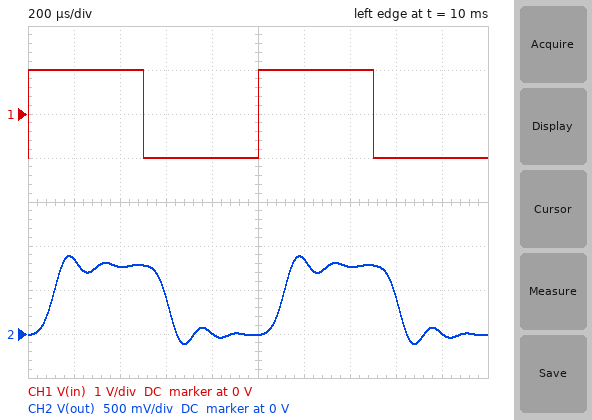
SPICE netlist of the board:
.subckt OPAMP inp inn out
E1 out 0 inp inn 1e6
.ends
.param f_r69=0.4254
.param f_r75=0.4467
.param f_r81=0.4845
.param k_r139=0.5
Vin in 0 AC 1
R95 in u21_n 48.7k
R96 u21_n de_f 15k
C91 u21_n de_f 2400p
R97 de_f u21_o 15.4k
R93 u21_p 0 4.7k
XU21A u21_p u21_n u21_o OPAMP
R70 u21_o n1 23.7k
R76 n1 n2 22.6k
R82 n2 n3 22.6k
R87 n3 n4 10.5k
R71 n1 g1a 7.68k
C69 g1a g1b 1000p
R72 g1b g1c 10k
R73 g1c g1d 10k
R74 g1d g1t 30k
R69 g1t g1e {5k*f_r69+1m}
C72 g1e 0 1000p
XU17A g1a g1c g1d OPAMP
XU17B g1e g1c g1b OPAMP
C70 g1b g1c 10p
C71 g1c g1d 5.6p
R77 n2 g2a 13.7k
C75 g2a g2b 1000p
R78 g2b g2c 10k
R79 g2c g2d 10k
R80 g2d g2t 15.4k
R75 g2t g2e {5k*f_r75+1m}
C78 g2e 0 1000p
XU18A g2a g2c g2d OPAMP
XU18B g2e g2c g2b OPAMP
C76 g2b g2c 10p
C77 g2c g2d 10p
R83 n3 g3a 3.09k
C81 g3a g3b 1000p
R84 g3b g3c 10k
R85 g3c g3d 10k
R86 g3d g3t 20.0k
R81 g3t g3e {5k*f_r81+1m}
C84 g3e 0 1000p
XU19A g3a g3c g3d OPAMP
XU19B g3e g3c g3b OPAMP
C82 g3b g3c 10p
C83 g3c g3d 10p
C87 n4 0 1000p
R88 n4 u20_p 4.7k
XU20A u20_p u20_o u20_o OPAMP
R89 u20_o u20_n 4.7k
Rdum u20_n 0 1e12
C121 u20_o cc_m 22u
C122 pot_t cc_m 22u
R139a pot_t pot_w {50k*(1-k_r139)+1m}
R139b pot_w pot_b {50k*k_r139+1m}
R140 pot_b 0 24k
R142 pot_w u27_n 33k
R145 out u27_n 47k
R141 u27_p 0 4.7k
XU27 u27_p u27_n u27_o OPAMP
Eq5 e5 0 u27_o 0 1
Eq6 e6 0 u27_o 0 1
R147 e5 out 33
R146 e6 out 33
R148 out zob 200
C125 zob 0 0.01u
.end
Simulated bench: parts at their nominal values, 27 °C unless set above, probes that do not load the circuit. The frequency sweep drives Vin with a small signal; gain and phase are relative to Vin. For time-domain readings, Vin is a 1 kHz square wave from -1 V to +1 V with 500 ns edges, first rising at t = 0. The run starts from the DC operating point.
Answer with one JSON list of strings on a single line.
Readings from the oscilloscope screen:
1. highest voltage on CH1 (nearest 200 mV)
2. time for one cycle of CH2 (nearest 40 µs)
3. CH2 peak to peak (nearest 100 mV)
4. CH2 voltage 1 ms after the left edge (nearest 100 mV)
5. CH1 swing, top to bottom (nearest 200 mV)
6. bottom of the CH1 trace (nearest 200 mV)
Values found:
["1.0 V", "1.00 ms", "1.0 V", "0 V", "2.0 V", "-1.0 V"]
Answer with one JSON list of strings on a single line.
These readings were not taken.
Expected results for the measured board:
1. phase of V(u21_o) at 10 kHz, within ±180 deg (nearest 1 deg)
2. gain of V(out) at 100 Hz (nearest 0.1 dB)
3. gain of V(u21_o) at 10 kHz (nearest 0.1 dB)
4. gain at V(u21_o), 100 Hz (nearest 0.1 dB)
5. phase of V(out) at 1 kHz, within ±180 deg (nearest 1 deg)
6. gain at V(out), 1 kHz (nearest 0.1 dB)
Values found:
["163 deg", "-8.1 dB", "-8.3 dB", "-4.1 dB", "-35 deg", "-8.3 dB"]
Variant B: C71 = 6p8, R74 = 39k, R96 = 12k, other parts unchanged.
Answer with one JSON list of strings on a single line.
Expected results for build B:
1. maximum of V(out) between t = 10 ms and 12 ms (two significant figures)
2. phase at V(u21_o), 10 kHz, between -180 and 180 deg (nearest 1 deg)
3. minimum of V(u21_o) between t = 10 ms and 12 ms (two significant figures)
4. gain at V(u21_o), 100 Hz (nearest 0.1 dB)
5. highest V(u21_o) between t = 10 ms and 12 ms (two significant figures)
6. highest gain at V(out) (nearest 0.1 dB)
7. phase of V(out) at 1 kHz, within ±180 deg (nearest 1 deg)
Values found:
["860 mV", "164 deg", "-560 mV", "-5.0 dB", "560 mV", "-7.3 dB", "-33 deg"]
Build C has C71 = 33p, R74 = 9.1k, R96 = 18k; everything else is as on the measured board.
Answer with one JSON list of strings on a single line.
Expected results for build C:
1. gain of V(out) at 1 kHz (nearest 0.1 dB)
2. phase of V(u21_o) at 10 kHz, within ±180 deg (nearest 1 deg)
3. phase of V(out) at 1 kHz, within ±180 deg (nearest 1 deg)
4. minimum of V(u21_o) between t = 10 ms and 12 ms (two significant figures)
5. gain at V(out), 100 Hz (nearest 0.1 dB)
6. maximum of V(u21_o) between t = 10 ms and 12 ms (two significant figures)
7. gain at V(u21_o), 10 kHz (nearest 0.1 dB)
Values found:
["-7.7 dB", "162 deg", "-36 deg", "-690 mV", "-7.3 dB", "690 mV", "-8.4 dB"]
